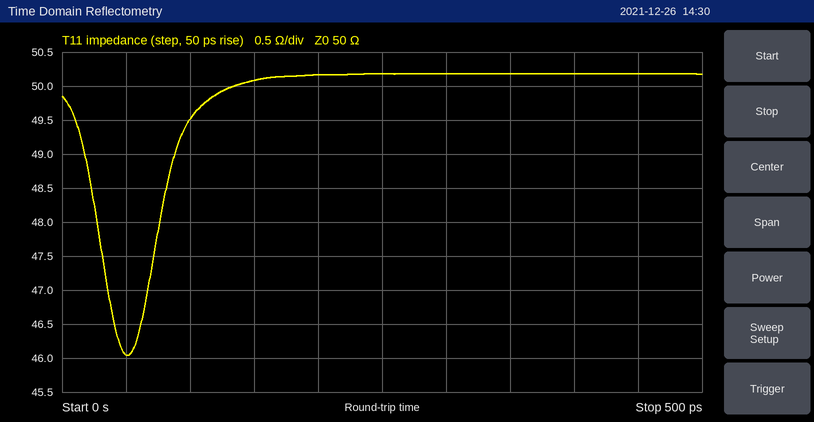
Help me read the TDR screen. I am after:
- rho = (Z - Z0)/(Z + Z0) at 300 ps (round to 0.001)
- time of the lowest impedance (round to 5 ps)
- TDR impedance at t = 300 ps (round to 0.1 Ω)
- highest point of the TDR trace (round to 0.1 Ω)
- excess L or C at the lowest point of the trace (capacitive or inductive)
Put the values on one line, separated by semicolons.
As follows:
+0.002; 50 ps; 50.2 Ω; 50.2 Ω; capacitive
